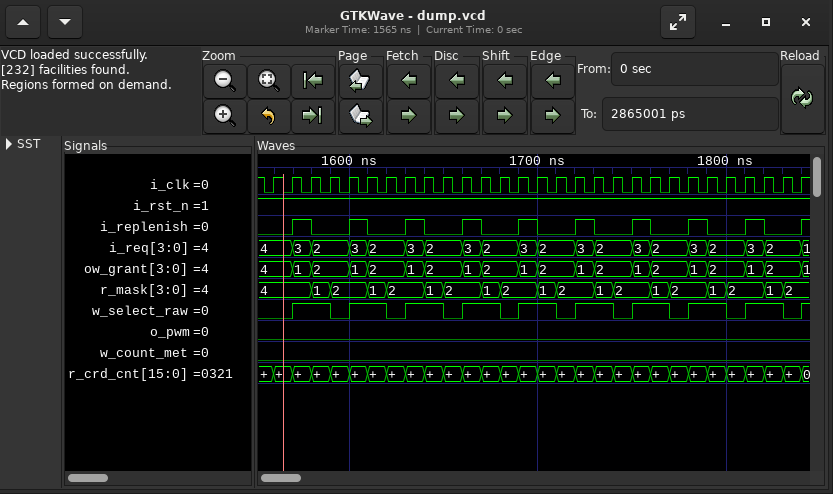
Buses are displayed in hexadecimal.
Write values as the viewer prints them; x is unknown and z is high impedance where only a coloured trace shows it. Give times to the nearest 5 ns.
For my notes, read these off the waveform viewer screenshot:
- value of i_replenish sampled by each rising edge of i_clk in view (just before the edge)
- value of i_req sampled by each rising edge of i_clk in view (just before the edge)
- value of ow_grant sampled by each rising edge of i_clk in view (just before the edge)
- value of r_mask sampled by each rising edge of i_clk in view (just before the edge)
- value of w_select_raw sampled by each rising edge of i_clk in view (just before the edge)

0 0 1 0 0 1 0 0 1 0 0 1 0 0 1 0 0 1 0 0 1 0 0 1 0 0 1 0 0
4, 4, 3, 2, 2, 3, 2, 2, 3, 2, 2, 3, 2, 2, 3, 2, 2, 3, 2, 2, 3, 2, 2, 3, 2, 2, 3, 2, 2
4, 4, 1, 2, 2, 1, 2, 2, 1, 2, 2, 1, 2, 2, 1, 2, 2, 1, 2, 2, 1, 2, 2, 1, 2, 2, 1, 2, 2
4, 4, 4, 1, 2, 2, 1, 2, 2, 1, 2, 2, 1, 2, 2, 1, 2, 2, 1, 2, 2, 1, 2, 2, 1, 2, 2, 1, 2
0 0 1 1 0 1 1 0 1 1 0 1 1 0 1 1 0 1 1 0 1 1 0 1 1 0 1 1 0
